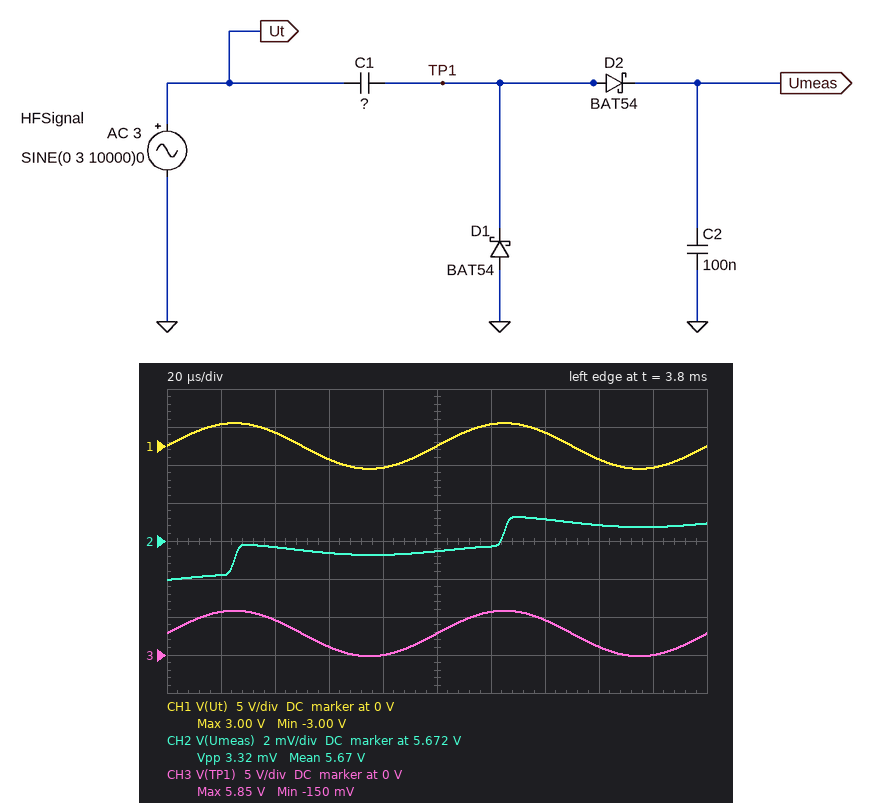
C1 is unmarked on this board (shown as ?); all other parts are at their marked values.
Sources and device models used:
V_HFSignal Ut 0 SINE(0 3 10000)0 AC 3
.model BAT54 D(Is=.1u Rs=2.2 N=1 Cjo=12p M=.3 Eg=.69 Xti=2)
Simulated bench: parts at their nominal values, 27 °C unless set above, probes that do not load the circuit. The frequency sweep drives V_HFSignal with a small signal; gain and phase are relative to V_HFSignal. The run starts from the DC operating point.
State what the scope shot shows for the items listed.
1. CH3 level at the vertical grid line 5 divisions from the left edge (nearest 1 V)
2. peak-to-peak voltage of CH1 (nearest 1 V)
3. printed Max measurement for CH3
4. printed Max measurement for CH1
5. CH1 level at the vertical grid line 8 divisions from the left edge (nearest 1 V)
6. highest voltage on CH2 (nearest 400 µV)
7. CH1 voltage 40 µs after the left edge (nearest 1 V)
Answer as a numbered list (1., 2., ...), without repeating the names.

1. 3 V
2. 6 V
3. 5.85 V
4. 3.00 V
5. -2 V
6. 5.6732 V
7. 2 V
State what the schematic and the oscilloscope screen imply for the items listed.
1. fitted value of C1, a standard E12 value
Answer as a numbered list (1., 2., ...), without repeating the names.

1. 150 nF
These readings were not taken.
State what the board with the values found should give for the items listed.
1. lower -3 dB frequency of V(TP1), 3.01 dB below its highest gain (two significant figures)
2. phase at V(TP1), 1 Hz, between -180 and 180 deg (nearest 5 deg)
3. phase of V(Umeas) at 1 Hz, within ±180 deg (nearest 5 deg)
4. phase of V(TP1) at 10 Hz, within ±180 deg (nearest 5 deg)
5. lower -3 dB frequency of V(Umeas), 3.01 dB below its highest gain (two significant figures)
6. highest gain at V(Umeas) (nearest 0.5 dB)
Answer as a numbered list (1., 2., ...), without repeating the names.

1. 9.3 Hz
2. 70 deg
3. 60 deg
4. 30 deg
5. 1.6 Hz
6. -7.5 dB
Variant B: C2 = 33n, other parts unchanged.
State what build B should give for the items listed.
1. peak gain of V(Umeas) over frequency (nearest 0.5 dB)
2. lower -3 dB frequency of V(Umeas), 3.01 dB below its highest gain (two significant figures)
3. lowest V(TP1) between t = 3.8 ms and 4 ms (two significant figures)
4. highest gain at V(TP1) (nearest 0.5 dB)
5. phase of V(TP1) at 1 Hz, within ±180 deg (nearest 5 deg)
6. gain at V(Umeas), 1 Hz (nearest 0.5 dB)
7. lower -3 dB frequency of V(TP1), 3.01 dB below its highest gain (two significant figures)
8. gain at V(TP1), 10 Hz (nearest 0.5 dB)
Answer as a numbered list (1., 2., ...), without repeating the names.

1. -3.0 dB
2. 2.6 Hz
3. -160 mV
4. 0 dB
5. 75 deg
6. -12.5 dB
7. 6.0 Hz
8. -2.0 dB
